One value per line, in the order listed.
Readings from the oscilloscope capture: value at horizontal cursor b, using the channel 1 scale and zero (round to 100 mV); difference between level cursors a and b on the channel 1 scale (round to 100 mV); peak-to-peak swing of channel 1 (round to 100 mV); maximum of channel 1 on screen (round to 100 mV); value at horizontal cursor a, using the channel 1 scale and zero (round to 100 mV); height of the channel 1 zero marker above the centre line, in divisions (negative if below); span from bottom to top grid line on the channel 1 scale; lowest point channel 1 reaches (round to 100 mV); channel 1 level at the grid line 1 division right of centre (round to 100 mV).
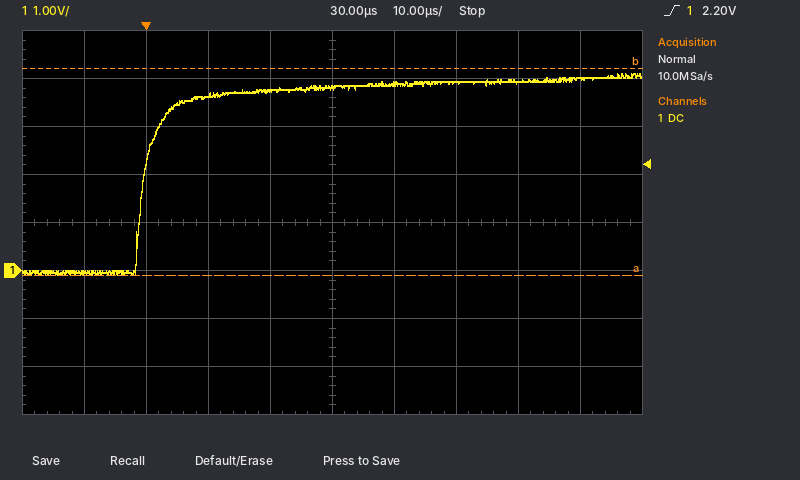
4.2 V
4.3 V
4.2 V
4.1 V
-100 mV
-1.0 div
8 V
-100 mV
3.9 V
